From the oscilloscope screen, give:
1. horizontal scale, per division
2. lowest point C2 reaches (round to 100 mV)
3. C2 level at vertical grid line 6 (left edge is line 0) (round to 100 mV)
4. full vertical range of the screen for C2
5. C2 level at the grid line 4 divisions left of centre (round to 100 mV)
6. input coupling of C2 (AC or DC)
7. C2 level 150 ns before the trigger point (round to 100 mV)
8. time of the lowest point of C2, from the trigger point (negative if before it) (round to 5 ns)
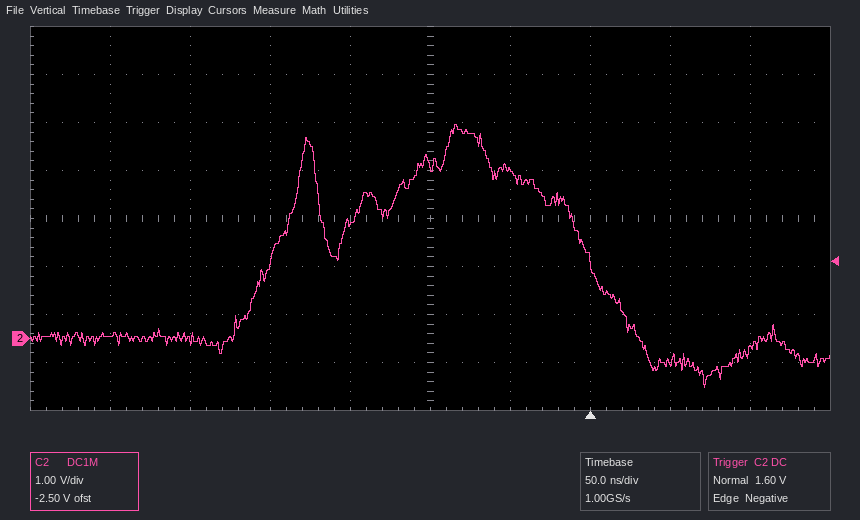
50 ns
-1.0 V
3.5 V
8 V
100 mV
DC
2.4 V
+70 ns
